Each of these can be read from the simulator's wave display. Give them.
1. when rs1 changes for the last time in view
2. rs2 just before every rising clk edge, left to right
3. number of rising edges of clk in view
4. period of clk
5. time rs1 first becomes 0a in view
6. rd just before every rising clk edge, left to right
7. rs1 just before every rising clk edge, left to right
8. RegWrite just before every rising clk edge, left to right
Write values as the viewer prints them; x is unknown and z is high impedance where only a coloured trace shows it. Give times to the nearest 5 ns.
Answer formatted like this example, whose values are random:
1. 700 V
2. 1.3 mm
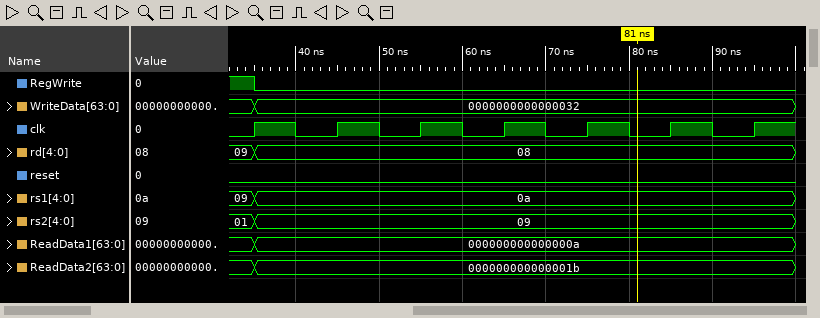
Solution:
1. 35 ns
2. 01, 09, 09, 09, 09, 09, 09
3. 7
4. 10 ns
5. 35 ns
6. 09, 08, 08, 08, 08, 08, 08
7. 09, 0a, 0a, 0a, 0a, 0a, 0a
8. 1 0 0 0 0 0 0
